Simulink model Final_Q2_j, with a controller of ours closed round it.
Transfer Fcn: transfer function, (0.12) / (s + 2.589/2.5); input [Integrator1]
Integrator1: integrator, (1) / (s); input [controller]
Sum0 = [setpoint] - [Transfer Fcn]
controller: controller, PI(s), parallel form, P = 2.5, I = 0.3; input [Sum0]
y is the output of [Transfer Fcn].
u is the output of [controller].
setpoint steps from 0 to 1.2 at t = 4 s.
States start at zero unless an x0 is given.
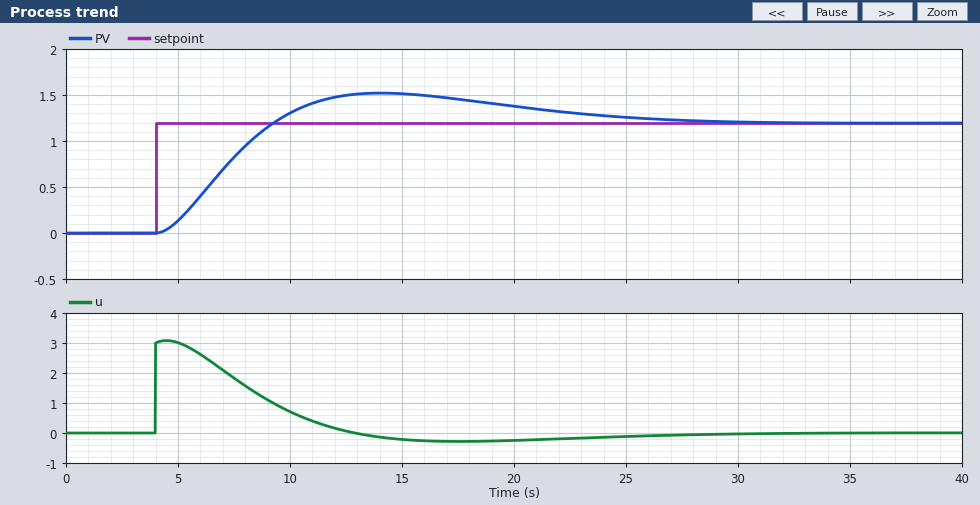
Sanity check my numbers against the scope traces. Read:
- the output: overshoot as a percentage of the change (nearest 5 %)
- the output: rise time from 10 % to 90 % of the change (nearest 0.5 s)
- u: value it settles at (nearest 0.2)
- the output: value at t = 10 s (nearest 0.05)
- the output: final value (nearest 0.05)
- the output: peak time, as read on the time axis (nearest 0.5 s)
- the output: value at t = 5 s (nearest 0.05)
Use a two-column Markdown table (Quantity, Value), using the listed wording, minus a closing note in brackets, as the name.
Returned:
| Quantity | Value |
|---|---|
| the output: overshoot as a percentage of the change | 25 % |
| the output: rise time from 10 % to 90 % of the change | 3.5 s |
| u: value it settles at | 0.0 |
| the output: value at t = 10 s | 1.30 |
| the output: final value | 1.20 |
| the output: peak time, as read on the time axis | 14.0 s |
| the output: value at t = 5 s | 0.15 |
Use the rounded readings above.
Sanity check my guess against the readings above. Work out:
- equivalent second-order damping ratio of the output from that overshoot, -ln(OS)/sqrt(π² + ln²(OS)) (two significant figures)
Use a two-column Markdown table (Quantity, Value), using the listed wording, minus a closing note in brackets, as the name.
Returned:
| Quantity | Value |
|---|---|
| equivalent second-order damping ratio of the output from that overshoot, -ln(OS)/sqrt(π² + ln²(OS)) | 0.40 |
